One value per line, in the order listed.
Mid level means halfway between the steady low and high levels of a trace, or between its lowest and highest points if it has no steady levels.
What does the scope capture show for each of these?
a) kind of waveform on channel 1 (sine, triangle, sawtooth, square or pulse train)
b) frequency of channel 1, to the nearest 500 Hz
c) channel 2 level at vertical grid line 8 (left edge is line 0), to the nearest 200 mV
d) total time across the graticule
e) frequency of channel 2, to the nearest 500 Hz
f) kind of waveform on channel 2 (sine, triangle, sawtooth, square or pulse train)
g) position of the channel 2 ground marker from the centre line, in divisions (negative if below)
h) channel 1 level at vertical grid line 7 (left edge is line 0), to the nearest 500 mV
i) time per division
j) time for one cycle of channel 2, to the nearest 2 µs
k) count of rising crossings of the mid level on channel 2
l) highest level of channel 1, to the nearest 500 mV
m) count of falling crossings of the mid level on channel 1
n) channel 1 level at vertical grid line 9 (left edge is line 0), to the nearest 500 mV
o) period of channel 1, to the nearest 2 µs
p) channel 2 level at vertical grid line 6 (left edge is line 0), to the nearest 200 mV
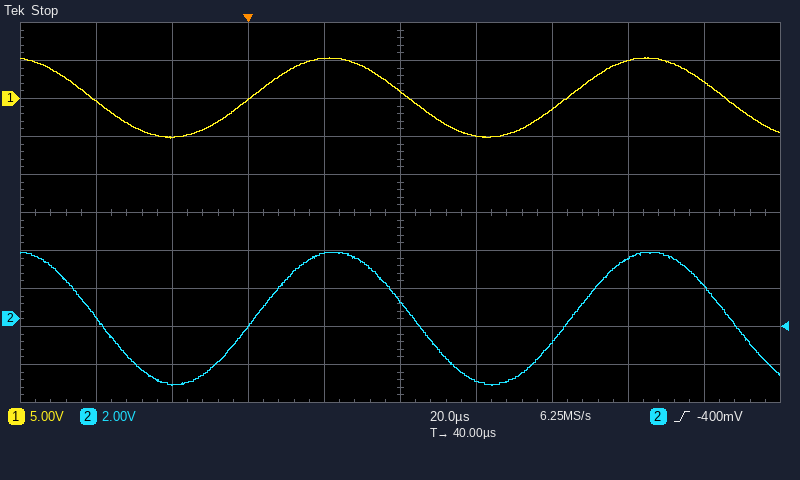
sine
12.0 kHz
3.2 V
200 µs
12.0 kHz
sine
-2.8 div
-1.5 V
20 µs
84 µs
2
5.5 V
3
2.0 V
84 µs
-3.2 V
